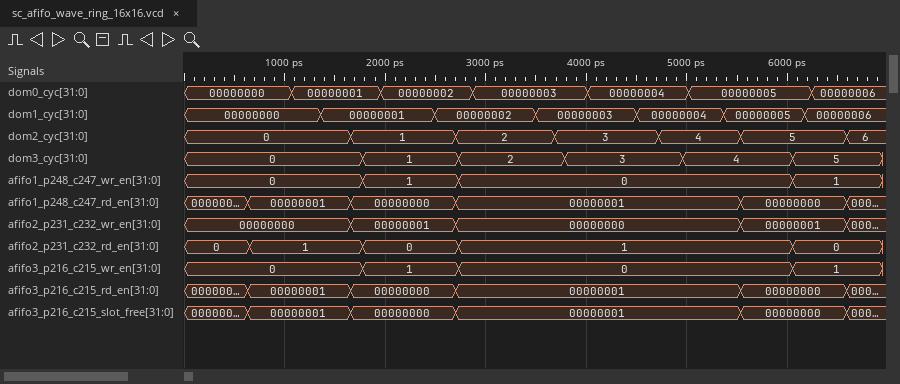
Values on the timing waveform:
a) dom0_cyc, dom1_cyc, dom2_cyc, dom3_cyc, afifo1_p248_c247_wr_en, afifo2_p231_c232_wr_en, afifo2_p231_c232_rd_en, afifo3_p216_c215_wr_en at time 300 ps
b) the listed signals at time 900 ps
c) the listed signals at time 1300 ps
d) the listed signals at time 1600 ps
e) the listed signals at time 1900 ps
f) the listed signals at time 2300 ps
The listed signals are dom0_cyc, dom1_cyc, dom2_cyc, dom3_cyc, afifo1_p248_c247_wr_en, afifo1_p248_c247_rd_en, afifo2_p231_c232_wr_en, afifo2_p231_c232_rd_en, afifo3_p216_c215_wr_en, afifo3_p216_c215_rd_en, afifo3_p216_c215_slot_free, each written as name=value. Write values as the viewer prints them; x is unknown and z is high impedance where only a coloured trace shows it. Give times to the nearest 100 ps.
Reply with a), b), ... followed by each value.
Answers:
a) dom0_cyc=00000000, dom1_cyc=00000000, dom2_cyc=0, dom3_cyc=0, afifo1_p248_c247_wr_en=0, afifo2_p231_c232_wr_en=00000000, afifo2_p231_c232_rd_en=0, afifo3_p216_c215_wr_en=0
b) dom0_cyc=00000000, dom1_cyc=00000000, dom2_cyc=0, dom3_cyc=0, afifo1_p248_c247_wr_en=0, afifo1_p248_c247_rd_en=00000001, afifo2_p231_c232_wr_en=00000000, afifo2_p231_c232_rd_en=1, afifo3_p216_c215_wr_en=0, afifo3_p216_c215_rd_en=00000001, afifo3_p216_c215_slot_free=00000001
c) dom0_cyc=00000001, dom1_cyc=00000000, dom2_cyc=0, dom3_cyc=0, afifo1_p248_c247_wr_en=0, afifo1_p248_c247_rd_en=00000001, afifo2_p231_c232_wr_en=00000000, afifo2_p231_c232_rd_en=1, afifo3_p216_c215_wr_en=0, afifo3_p216_c215_rd_en=00000001, afifo3_p216_c215_slot_free=00000001
d) dom0_cyc=00000001, dom1_cyc=00000001, dom2_cyc=0, dom3_cyc=0, afifo1_p248_c247_wr_en=0, afifo1_p248_c247_rd_en=00000001, afifo2_p231_c232_wr_en=00000000, afifo2_p231_c232_rd_en=1, afifo3_p216_c215_wr_en=0, afifo3_p216_c215_rd_en=00000001, afifo3_p216_c215_slot_free=00000001
e) dom0_cyc=00000001, dom1_cyc=00000001, dom2_cyc=1, dom3_cyc=1, afifo1_p248_c247_wr_en=1, afifo1_p248_c247_rd_en=00000000, afifo2_p231_c232_wr_en=00000001, afifo2_p231_c232_rd_en=0, afifo3_p216_c215_wr_en=1, afifo3_p216_c215_rd_en=00000000, afifo3_p216_c215_slot_free=00000000
f) dom0_cyc=00000002, dom1_cyc=00000001, dom2_cyc=1, dom3_cyc=1, afifo1_p248_c247_wr_en=1, afifo1_p248_c247_rd_en=00000000, afifo2_p231_c232_wr_en=00000001, afifo2_p231_c232_rd_en=0, afifo3_p216_c215_wr_en=1, afifo3_p216_c215_rd_en=00000000, afifo3_p216_c215_slot_free=00000000
